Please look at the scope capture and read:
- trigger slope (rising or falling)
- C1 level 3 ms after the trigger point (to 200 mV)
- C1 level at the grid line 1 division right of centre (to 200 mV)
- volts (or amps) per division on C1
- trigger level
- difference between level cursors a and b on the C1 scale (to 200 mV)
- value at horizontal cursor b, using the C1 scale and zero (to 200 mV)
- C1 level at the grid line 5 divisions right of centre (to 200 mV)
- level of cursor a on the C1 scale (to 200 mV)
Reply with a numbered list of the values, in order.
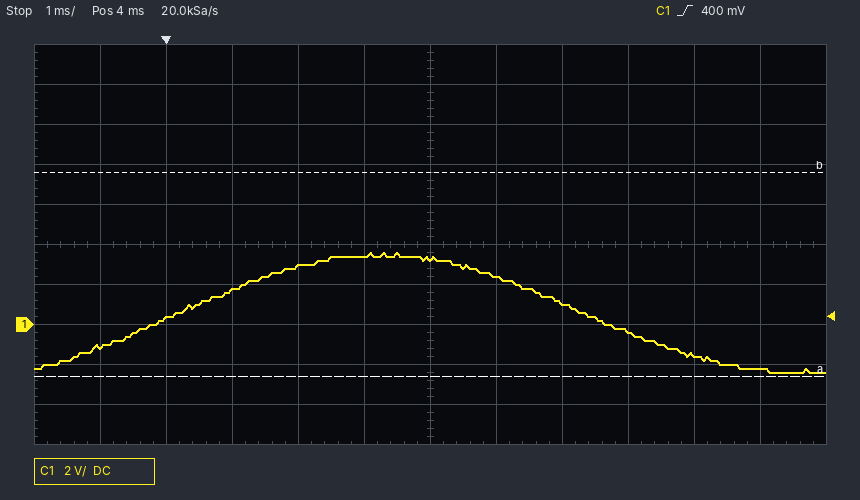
1. rising
2. 3.4 V
3. 2.4 V
4. 2 V
5. 400 mV
6. 10.2 V
7. 7.6 V
8. -2.2 V
9. -2.6 V
